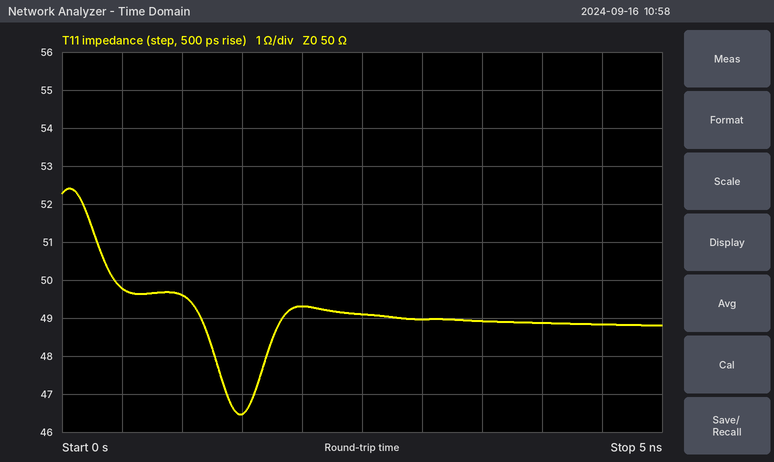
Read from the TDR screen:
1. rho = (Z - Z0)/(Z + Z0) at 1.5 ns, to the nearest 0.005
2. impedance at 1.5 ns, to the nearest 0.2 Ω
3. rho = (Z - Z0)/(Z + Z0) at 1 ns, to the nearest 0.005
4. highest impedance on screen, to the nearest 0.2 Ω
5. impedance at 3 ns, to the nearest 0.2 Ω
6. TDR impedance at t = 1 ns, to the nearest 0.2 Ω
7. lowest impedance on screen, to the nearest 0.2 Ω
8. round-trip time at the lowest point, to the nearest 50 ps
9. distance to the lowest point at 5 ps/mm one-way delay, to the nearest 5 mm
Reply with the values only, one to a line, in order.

-0.035
46.4 Ω
-0.005
52.4 Ω
49.0 Ω
49.6 Ω
46.4 Ω
1.50 ns
150 mm
